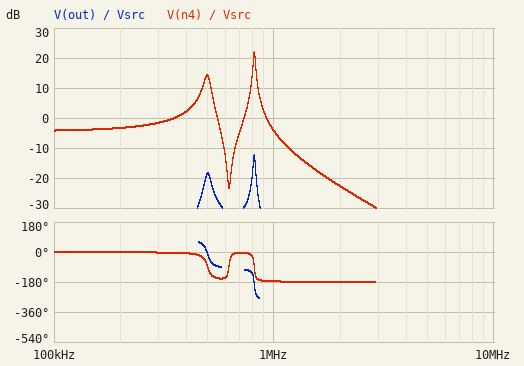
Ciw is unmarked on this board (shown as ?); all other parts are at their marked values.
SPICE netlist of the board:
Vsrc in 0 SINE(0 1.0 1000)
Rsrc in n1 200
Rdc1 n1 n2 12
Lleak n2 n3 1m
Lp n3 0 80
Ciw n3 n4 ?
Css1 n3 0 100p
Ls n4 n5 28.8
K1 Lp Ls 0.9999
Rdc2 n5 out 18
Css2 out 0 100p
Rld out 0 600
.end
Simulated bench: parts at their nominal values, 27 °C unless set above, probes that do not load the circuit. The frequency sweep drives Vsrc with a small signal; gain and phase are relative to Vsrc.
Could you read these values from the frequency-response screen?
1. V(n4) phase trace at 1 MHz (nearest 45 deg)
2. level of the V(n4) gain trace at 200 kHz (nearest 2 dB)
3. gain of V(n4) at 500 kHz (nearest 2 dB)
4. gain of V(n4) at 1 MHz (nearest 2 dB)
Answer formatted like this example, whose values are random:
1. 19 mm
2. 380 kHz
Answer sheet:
1. -180 deg
2. -4 dB
3. 14 dB
4. -4 dB
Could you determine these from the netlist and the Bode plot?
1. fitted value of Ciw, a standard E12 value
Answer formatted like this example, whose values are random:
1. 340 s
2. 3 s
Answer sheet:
1. 6.8 pF
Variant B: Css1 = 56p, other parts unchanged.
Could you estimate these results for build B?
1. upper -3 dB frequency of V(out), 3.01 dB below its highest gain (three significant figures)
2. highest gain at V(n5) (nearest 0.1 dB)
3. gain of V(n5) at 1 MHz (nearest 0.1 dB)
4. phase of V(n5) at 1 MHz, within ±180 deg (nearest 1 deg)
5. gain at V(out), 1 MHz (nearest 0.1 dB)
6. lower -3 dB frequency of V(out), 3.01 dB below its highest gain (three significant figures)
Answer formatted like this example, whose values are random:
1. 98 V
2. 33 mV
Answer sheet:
1. 837 kHz
2. -3.7 dB
3. -35.8 dB
4. 76 deg
5. -36.1 dB
6. 819 kHz
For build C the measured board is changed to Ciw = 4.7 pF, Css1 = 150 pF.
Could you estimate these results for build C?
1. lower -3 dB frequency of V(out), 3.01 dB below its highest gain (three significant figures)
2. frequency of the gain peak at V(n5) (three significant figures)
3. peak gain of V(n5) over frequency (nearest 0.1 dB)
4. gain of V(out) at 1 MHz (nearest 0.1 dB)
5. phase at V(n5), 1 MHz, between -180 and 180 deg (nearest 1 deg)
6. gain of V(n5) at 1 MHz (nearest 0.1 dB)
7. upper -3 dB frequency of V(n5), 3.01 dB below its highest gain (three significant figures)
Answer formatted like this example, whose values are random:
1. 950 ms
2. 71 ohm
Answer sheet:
1. 965 kHz
2. 973 kHz
3. -20.8 dB
4. -32.8 dB
5. 88 deg
6. -32.6 dB
7. 980 kHz
